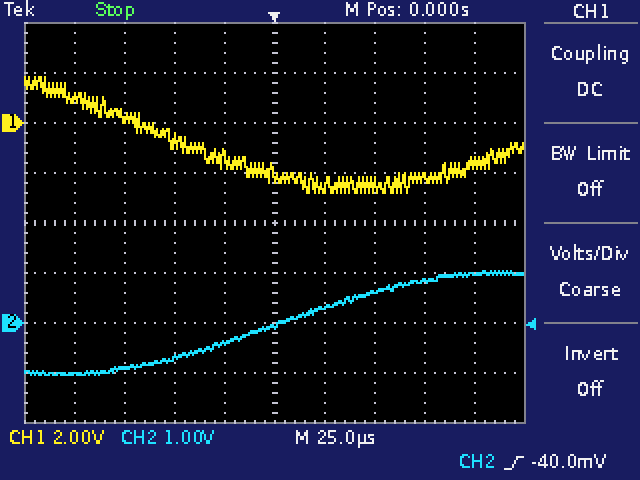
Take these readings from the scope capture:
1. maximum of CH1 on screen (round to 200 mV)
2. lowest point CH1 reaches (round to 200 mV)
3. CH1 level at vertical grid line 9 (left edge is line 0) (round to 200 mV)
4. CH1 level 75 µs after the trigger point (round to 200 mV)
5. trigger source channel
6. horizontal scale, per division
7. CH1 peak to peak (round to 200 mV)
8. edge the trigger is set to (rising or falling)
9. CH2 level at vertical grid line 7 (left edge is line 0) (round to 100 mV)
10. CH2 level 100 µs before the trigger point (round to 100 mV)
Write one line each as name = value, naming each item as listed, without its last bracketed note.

maximum of CH1 on screen = 1.8 V
lowest point CH1 reaches = -2.8 V
CH1 level at vertical grid line 9 (left edge is line 0) = -1.6 V
CH1 level 75 µs after the trigger point = -2.2 V
trigger source channel = CH2
horizontal scale, per division = 25 µs
CH1 peak to peak = 4.6 V
edge the trigger is set to = rising
CH2 level at vertical grid line 7 (left edge is line 0) = 600 mV
CH2 level 100 µs before the trigger point = -1.0 V
